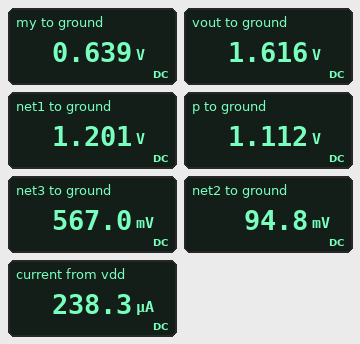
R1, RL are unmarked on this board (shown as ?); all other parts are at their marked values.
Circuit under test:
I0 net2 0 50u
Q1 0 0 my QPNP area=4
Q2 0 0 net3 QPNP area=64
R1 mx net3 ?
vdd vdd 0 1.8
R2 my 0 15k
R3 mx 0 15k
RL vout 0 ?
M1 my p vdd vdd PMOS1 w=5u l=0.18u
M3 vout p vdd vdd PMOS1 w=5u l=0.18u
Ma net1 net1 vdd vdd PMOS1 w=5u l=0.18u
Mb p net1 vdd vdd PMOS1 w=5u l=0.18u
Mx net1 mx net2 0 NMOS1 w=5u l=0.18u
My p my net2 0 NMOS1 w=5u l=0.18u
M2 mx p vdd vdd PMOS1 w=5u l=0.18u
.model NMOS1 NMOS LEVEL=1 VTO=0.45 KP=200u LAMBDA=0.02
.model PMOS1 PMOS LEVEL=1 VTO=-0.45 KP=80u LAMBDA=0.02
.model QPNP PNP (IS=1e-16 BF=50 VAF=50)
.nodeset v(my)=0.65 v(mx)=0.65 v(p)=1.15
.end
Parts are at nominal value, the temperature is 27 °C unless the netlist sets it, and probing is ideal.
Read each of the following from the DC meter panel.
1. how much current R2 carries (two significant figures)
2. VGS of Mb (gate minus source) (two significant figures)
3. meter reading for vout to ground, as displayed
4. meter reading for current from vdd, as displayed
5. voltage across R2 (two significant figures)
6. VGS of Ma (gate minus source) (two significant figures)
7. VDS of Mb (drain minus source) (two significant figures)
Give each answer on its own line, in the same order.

43 µA
-600 mV
1.616 V
238.3 µA
640 mV
-600 mV
-690 mV
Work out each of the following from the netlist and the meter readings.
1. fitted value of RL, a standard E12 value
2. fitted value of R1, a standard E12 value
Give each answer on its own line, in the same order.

27 kΩ
3.3 kΩ
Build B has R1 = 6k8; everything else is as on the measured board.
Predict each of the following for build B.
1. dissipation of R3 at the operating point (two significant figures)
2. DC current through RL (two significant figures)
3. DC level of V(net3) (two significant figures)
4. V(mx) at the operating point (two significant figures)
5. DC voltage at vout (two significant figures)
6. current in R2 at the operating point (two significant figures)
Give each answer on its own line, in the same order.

26 µW
51 µA
550 mV
620 mV
1.4 V
41 µA
